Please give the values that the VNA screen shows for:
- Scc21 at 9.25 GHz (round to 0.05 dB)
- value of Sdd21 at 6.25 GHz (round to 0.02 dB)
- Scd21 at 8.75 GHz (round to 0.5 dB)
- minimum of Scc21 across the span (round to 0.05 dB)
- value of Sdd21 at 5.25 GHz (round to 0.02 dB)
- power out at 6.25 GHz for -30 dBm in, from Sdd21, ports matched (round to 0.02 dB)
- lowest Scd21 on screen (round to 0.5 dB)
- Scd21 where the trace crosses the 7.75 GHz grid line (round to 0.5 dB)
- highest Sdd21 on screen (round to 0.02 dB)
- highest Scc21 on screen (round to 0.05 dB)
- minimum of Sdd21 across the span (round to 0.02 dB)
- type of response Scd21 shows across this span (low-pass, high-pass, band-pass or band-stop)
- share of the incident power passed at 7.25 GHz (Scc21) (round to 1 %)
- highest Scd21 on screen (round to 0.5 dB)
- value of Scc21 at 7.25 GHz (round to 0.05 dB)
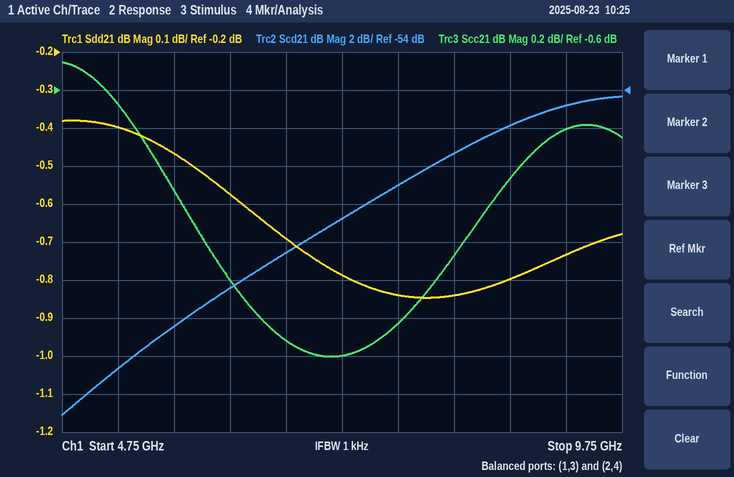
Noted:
-0.80 dB
-0.58 dB
-56.0 dB
-2.00 dB
-0.40 dB
-30.58 dBm
-71.0 dB
-59.0 dB
-0.38 dB
-0.45 dB
-0.84 dB
high-pass
63 %
-54.5 dB
-2.00 dB
